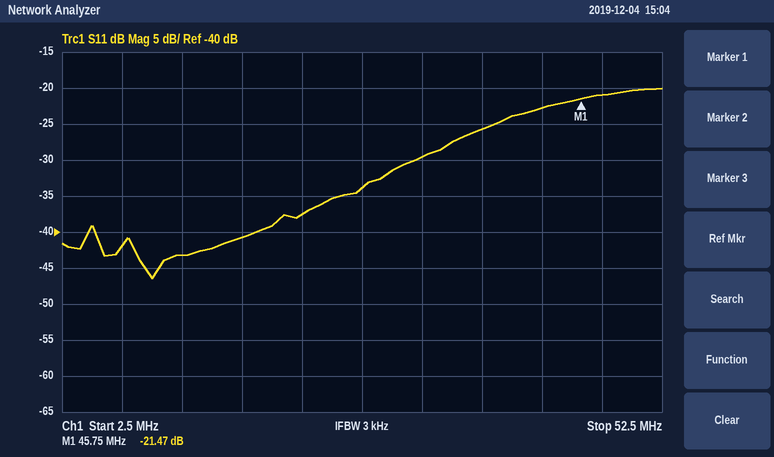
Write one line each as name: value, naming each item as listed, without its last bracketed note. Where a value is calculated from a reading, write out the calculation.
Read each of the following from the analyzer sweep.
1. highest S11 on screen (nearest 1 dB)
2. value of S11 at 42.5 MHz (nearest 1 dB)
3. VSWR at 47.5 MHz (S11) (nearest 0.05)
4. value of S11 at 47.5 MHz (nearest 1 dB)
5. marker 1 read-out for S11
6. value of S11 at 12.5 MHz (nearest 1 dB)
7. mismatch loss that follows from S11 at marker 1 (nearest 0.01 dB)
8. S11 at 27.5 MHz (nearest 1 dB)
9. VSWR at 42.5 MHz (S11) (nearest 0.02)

highest S11 on screen: -20 dB
value of S11 at 42.5 MHz: -23 dB
VSWR at 47.5 MHz (S11): |Γ| = 10^(-21/20) = 0.0891; VSWR = (1 + 0.0891)/(1 − 0.0891) ≈ 1.20
value of S11 at 47.5 MHz: -21 dB
marker 1 read-out for S11: -21.47 dB
value of S11 at 12.5 MHz: -43 dB
mismatch loss that follows from S11 at marker 1: −10 log10(1 − 10^(-21.47/10)) ≈ 0.03 dB
S11 at 27.5 MHz: -34 dB
VSWR at 42.5 MHz (S11): |Γ| = 10^(-23/20) = 0.0708; VSWR = (1 + 0.0708)/(1 − 0.0708) ≈ 1.15, so 1.16 to the nearest 0.02
